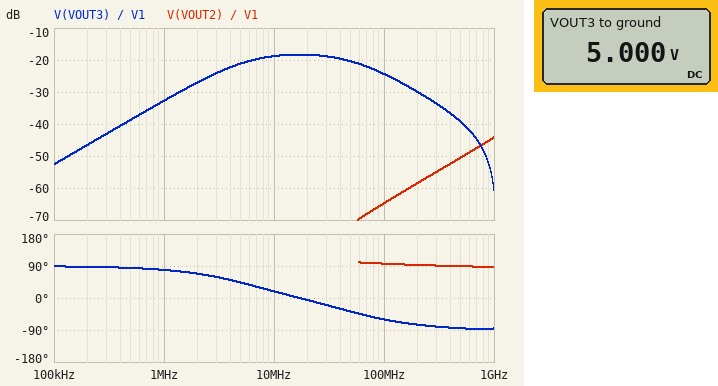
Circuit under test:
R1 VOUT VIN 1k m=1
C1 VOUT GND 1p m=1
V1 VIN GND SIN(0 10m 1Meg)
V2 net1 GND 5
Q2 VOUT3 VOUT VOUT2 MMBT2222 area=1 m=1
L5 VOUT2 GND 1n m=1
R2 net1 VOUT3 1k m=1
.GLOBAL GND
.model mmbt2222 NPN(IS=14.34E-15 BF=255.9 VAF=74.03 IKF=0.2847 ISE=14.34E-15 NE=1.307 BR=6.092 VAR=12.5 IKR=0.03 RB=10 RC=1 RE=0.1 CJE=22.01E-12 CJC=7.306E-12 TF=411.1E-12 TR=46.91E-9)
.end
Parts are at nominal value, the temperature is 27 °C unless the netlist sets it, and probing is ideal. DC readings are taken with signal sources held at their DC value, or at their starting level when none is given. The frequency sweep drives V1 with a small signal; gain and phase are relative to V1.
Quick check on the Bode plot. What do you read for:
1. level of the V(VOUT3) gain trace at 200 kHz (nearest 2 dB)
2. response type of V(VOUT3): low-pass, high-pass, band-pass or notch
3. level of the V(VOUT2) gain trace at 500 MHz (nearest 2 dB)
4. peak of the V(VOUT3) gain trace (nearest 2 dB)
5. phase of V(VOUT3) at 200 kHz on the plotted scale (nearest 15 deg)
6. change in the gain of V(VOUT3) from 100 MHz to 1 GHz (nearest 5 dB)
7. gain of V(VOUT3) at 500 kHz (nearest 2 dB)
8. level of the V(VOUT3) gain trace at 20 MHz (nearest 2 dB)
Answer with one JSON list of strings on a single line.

["-46 dB", "band-pass", "-50 dB", "-18 dB", "90 deg", "-35 dB", "-38 dB", "-18 dB"]
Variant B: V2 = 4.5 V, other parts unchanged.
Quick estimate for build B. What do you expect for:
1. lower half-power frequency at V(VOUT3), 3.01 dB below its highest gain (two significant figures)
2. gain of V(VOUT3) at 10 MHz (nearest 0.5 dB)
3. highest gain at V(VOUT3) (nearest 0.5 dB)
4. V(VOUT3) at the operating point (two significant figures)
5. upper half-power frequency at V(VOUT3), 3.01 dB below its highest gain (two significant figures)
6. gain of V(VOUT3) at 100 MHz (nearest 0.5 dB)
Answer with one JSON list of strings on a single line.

["4.7 MHz", "-18.5 dB", "-18.0 dB", "4.5 V", "60 MHz", "-24.5 dB"]
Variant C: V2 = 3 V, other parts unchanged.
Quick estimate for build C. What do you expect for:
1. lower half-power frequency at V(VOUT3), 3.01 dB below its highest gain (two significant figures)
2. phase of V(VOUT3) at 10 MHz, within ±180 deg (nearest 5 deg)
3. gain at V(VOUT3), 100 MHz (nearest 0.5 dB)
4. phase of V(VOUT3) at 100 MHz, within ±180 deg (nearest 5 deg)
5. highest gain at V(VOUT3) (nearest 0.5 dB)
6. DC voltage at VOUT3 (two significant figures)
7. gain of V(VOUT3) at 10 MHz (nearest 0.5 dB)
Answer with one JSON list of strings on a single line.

["4.6 MHz", "15 deg", "-24.0 dB", "-65 deg", "-17.5 dB", "3.0 V", "-18.0 dB"]
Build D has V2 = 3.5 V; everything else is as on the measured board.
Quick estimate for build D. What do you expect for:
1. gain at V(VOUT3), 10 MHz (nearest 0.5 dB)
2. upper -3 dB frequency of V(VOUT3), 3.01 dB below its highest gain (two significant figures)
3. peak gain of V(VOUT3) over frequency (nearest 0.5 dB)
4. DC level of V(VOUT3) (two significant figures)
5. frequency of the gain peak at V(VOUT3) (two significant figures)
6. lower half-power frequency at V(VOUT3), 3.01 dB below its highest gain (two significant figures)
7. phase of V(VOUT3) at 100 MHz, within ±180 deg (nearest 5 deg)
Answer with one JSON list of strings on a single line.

["-18.0 dB", "57 MHz", "-17.5 dB", "3.5 V", "16 MHz", "4.6 MHz", "-60 deg"]
